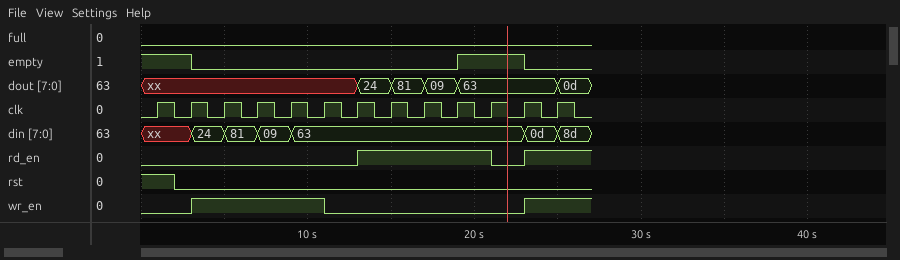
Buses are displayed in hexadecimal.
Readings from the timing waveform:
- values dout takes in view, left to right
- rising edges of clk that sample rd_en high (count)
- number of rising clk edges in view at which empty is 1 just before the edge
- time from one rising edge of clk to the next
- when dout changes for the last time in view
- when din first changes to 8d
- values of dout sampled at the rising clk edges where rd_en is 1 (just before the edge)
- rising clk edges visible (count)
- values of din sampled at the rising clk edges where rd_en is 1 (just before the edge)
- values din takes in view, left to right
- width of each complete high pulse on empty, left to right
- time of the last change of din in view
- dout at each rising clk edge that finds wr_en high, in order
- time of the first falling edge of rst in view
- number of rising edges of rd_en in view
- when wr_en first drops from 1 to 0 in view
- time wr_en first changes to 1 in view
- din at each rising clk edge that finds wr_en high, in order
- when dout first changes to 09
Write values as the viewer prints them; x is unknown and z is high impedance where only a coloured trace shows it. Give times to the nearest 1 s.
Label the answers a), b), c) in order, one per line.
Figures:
a) xx, 24, 81, 09, 63, 0d
b) 5
c) 4
d) 2 s
e) 25 s
f) 25 s
g) 24, 81, 09, 63, 63
h) 13
i) 63, 63, 63, 63, 0d
j) xx, 24, 81, 09, 63, 0d, 8d
k) 4 s
l) 25 s
m) xx, xx, xx, xx, 63
n) 2 s
o) 2
p) 11 s
q) 3 s
r) 24, 81, 09, 63, 0d
s) 17 s
